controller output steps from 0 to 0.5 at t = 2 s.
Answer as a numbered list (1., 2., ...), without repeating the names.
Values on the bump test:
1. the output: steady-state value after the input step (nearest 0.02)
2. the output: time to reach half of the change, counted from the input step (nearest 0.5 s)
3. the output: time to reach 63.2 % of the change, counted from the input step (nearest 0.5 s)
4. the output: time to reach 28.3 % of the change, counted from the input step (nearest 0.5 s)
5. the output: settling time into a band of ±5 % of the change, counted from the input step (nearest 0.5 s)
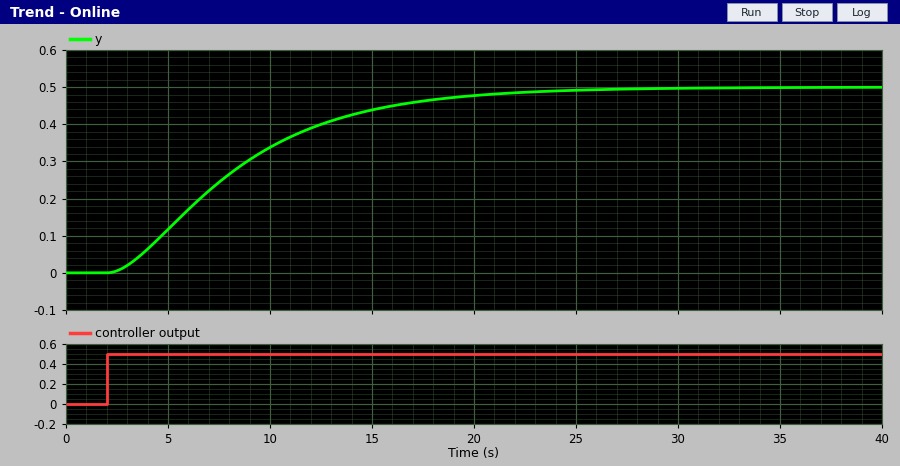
1. 0.50
2. 5.5 s
3. 7.5 s
4. 3.5 s
5. 17.5 s
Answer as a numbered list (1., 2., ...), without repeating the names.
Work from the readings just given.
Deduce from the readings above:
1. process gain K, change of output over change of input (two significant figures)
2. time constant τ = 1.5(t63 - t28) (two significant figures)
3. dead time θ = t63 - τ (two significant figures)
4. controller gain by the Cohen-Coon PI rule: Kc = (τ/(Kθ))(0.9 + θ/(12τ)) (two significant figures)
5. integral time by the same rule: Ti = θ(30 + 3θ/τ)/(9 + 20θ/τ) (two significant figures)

1. 1.0
2. 6.0 s
3. 1.5 s
4. 3.7
5. 3.3 s
